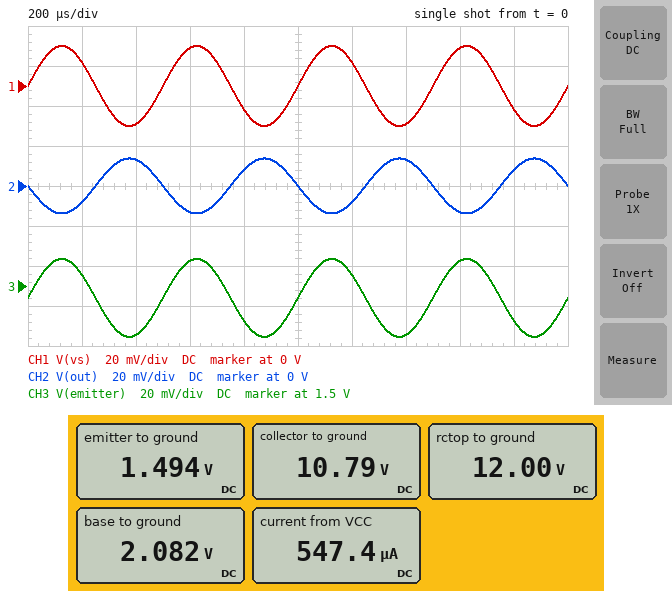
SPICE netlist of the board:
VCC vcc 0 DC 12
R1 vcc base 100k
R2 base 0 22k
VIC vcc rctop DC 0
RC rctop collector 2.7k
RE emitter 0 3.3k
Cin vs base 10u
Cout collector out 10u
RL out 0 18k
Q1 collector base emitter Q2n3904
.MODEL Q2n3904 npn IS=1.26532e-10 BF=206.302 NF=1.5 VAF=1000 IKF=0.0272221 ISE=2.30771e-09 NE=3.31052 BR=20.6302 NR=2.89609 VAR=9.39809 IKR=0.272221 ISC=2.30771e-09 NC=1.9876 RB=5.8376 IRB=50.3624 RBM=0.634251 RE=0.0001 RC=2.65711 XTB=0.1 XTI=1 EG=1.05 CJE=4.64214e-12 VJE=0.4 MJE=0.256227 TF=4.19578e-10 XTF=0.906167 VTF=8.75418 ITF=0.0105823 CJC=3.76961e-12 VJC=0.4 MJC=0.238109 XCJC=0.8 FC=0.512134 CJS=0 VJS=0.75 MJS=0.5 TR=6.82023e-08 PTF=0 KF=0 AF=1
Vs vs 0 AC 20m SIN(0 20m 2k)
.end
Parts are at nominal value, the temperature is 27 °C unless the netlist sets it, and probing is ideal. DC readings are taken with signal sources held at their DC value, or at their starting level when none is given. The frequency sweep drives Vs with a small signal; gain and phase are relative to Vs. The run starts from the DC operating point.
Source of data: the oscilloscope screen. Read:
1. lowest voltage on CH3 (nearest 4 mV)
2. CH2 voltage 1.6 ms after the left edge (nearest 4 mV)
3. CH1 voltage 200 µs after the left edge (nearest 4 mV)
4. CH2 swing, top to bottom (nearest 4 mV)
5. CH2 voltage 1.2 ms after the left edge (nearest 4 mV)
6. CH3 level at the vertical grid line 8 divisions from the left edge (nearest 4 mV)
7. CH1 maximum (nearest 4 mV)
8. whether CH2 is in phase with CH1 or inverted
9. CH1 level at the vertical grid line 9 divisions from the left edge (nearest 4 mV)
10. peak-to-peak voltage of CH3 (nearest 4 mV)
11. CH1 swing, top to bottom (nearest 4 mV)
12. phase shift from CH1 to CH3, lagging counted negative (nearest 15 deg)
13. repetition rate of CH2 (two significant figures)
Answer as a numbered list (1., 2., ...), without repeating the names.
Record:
1. 1.476 V
2. -12 mV
3. 12 mV
4. 28 mV
5. -8 mV
6. 1.512 V
7. 20 mV
8. inverted
9. -12 mV
10. 40 mV
11. 40 mV
12. 0 deg
13. 2.0 kHz
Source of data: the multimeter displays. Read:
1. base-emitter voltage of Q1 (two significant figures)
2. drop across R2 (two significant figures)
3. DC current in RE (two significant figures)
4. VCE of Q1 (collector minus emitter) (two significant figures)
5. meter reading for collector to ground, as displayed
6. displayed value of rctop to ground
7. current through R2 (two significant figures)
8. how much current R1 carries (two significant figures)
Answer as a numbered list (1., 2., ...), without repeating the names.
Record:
1. 590 mV
2. 2.1 V
3. 450 µA
4. 9.3 V
5. 10.79 V
6. 12.00 V
7. 95 µA
8. 99 µA
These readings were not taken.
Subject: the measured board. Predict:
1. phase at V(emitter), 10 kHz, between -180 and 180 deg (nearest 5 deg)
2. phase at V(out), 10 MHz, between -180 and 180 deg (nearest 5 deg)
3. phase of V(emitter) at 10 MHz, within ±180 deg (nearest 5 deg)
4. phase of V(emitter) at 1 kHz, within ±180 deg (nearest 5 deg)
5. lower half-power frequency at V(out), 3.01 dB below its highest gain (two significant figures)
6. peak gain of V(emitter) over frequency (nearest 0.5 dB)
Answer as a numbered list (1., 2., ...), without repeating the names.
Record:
1. 0 deg
2. 140 deg
3. 0 deg
4. 0 deg
5. 13 MHz
6. 0 dB
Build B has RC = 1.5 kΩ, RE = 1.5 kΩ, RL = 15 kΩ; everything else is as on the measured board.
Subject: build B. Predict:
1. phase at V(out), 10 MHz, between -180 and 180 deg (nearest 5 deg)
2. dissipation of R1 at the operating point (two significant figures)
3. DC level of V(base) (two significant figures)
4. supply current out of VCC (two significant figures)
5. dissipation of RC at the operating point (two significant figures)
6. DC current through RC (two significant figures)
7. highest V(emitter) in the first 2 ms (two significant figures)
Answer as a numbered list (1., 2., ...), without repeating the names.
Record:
1. 160 deg
2. 1.0 mW
3. 2.0 V
4. 1.0 mA
5. 1.3 mW
6. 930 µA
7. 1.4 V
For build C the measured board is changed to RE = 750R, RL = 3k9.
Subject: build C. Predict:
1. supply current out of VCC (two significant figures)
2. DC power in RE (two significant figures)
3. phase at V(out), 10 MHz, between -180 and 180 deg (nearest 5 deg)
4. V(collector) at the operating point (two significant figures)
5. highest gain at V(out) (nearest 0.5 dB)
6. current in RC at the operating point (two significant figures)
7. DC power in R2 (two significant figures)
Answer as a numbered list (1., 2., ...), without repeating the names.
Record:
1. 1.8 mA
2. 2.2 mW
3. 160 deg
4. 7.4 V
5. 6.0 dB
6. 1.7 mA
7. 170 µW
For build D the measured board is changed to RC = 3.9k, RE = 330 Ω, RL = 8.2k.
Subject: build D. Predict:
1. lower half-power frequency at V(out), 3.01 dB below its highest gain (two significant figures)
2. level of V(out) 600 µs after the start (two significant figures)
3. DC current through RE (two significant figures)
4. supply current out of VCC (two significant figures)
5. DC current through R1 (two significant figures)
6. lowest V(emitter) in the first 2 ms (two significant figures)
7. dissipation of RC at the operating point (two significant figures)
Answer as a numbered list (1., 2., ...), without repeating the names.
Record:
1. 19 Hz
2. -54 mV
3. 2.8 mA
4. 2.9 mA
5. 100 µA
6. 910 mV
7. 30 mW
